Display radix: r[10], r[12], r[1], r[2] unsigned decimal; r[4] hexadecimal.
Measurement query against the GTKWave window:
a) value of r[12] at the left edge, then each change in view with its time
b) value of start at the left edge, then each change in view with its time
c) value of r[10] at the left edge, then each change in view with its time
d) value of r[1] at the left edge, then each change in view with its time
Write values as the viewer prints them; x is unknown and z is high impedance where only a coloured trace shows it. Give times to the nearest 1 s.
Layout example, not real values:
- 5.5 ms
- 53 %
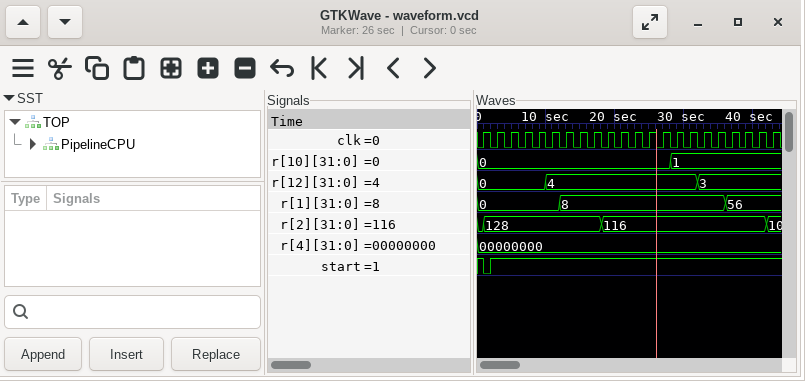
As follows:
- 0, 4 at 10 s, 3 at 32 s
- 1, 0 at 1 s, 1 at 2 s
- 0, 1 at 28 s
- 0, 8 at 12 s, 56 at 36 s
